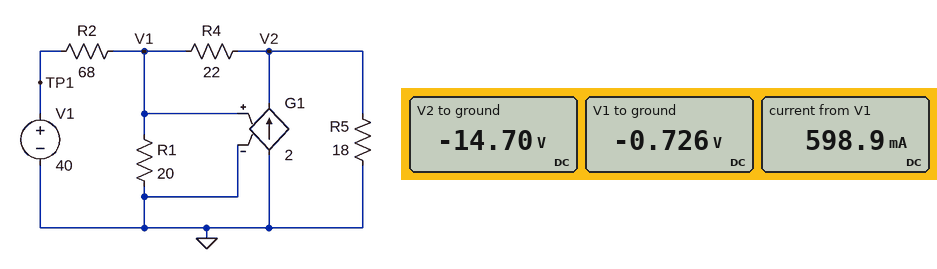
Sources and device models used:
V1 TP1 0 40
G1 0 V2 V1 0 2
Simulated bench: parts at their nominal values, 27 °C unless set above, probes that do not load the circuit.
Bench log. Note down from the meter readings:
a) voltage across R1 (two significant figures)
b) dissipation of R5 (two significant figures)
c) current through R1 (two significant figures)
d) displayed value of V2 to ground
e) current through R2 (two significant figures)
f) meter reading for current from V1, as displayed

730 mV
12 W
36 mA
-14.70 V
600 mA
598.9 mA
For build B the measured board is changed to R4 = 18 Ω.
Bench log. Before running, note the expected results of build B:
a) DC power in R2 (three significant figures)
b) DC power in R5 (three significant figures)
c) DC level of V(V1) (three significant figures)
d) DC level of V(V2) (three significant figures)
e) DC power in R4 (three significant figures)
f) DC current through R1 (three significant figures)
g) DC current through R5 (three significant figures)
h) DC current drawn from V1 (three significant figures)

24.3 W
7.99 W
-648 mV
-12.0 V
7.15 W
32.4 mA
666 mA
598 mA
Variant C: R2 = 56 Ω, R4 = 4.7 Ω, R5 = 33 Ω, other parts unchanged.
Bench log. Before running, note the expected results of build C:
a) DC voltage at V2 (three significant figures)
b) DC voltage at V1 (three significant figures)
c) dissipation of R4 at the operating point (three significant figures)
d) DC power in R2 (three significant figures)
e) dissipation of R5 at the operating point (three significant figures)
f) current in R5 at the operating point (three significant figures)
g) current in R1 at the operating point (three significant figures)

-3.93 V
-431 mV
2.60 W
29.2 W
467 mW
119 mA
21.6 mA
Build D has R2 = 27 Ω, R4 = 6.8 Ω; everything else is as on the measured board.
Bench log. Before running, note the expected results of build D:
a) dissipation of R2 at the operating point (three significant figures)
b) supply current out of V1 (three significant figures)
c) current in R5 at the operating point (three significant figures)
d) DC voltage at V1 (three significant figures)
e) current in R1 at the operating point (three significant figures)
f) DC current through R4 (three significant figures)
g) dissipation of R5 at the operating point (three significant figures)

62.6 W
1.52 A
659 mA
-1.12 V
55.9 mA
1.58 A
7.81 W
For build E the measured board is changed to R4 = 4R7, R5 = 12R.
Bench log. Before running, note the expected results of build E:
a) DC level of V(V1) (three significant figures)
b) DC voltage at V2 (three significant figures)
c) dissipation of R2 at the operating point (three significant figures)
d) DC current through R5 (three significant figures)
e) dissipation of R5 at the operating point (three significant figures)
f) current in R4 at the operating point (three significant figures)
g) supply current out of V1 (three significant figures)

-448 mV
-3.35 V
24.1 W
279 mA
935 mW
617 mA
595 mA
